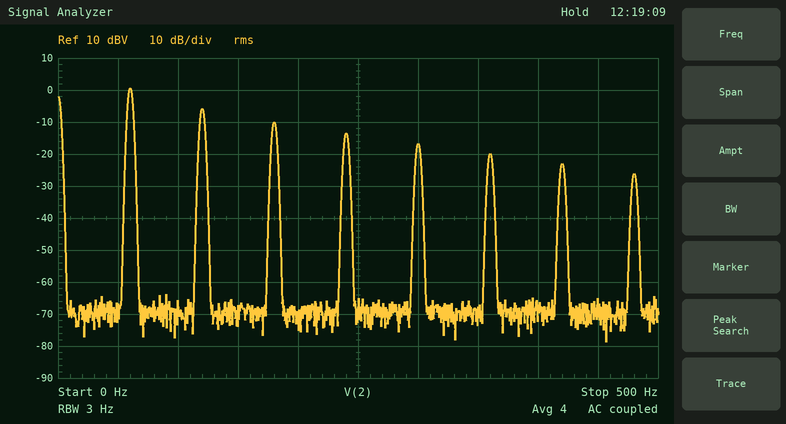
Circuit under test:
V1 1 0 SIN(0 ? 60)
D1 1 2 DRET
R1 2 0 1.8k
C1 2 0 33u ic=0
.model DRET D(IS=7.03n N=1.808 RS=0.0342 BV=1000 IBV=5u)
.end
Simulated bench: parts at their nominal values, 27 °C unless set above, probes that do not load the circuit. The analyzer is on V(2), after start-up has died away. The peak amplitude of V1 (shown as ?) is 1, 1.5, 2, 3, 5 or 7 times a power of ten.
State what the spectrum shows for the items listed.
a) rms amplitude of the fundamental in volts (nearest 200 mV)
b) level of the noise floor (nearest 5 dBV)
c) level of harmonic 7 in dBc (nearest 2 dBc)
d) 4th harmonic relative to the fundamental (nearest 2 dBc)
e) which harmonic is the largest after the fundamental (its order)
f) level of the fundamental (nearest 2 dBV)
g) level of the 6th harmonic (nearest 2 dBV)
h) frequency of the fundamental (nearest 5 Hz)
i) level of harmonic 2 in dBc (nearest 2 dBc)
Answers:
1.0 V
-70 dBV
-24 dBc
-14 dBc
2
0 dBV
-20 dBV
60 Hz
-6 dBc
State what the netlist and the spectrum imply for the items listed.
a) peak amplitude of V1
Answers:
20 V
